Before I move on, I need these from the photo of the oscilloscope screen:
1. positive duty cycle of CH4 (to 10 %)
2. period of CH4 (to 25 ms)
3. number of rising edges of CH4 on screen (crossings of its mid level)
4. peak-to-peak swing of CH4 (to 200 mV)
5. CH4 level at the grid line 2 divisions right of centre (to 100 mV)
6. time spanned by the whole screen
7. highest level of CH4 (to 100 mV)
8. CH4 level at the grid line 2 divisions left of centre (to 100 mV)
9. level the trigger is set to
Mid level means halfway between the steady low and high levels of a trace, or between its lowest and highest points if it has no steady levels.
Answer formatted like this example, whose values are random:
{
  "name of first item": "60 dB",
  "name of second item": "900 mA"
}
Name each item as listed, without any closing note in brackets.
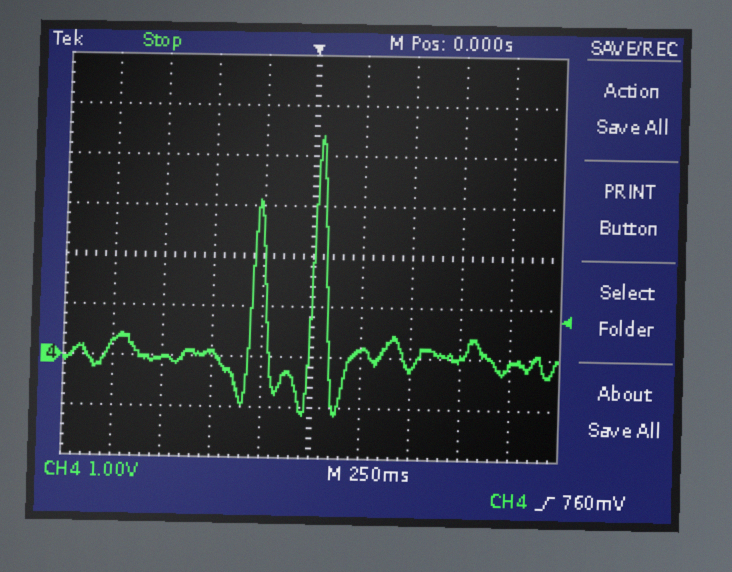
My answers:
{
  "positive duty cycle of CH4": "20 %",
  "period of CH4": "300 ms",
  "number of rising edges of CH4 on screen": "2",
  "peak-to-peak swing of CH4": "5.6 V",
  "CH4 level at the grid line 2 divisions right of centre": "-200 mV",
  "time spanned by the whole screen": "2.5 s",
  "highest level of CH4": "4.4 V",
  "CH4 level at the grid line 2 divisions left of centre": "100 mV",
  "level the trigger is set to": "760 mV"
}
